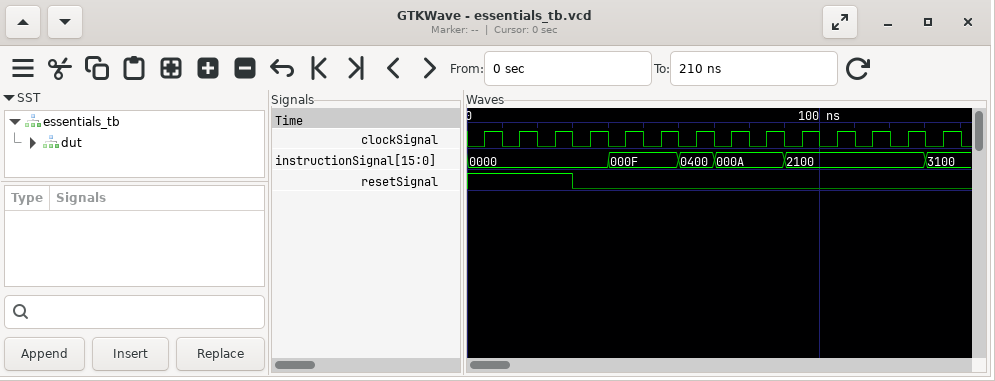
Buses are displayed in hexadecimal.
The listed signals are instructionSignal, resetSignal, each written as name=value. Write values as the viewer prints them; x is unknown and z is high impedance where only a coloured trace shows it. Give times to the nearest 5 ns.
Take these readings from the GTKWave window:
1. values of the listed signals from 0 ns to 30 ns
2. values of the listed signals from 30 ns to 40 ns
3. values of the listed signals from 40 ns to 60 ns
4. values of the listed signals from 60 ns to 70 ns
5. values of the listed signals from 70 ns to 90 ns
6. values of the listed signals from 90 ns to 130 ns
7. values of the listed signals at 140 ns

instructionSignal=0000, resetSignal=1
instructionSignal=0000, resetSignal=0
instructionSignal=000F, resetSignal=0
instructionSignal=0400, resetSignal=0
instructionSignal=000A, resetSignal=0
instructionSignal=2100, resetSignal=0
instructionSignal=3100, resetSignal=0
